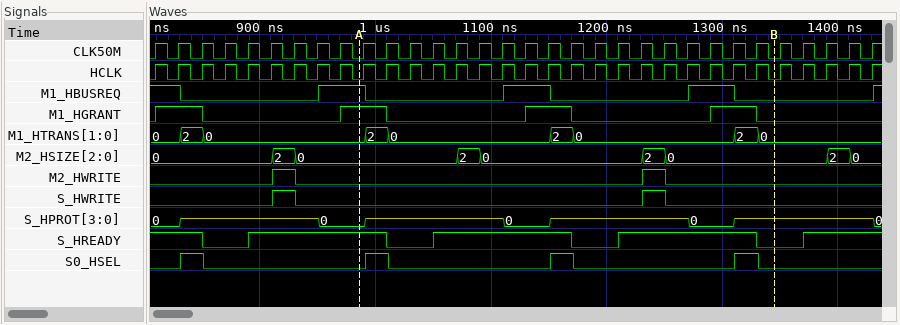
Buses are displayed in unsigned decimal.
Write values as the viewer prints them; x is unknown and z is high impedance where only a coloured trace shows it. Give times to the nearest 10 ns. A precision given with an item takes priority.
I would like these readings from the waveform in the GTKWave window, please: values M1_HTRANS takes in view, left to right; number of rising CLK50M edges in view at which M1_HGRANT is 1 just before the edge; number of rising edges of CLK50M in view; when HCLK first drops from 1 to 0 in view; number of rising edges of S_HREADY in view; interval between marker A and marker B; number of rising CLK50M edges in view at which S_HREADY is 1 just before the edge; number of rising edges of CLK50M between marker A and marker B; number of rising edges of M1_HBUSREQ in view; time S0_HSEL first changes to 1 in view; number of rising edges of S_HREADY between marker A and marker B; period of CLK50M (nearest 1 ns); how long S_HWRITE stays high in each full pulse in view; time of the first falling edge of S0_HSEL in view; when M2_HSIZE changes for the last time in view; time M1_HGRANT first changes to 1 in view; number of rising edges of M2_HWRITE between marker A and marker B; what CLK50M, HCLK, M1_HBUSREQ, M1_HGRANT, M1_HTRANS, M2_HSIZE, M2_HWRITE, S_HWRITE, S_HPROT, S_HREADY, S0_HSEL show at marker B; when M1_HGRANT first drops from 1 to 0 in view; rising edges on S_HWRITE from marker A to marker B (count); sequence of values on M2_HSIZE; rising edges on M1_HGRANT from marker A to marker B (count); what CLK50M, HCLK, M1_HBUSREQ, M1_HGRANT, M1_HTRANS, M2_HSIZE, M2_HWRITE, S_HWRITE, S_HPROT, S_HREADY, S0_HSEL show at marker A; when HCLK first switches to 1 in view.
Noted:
0, 2, 0, 2, 0, 2, 0, 2, 0
8
32
820 ns
4
360 ns
24
18
4
830 ns
2
20 ns
20 ns, 20 ns
850 ns
1410 ns
810 ns
1
CLK50M=0, HCLK=0, M1_HBUSREQ=0, M1_HGRANT=0, M1_HTRANS=0, M2_HSIZE=0, M2_HWRITE=0, S_HWRITE=0, S_HPROT=z, S_HREADY=0, S0_HSEL=0
850 ns
1
0, 2, 0, 2, 0, 2, 0, 2, 0
2
CLK50M=0, HCLK=0, M1_HBUSREQ=1, M1_HGRANT=1, M1_HTRANS=0, M2_HSIZE=0, M2_HWRITE=0, S_HWRITE=0, S_HPROT=0, S_HREADY=1, S0_HSEL=0
810 ns
